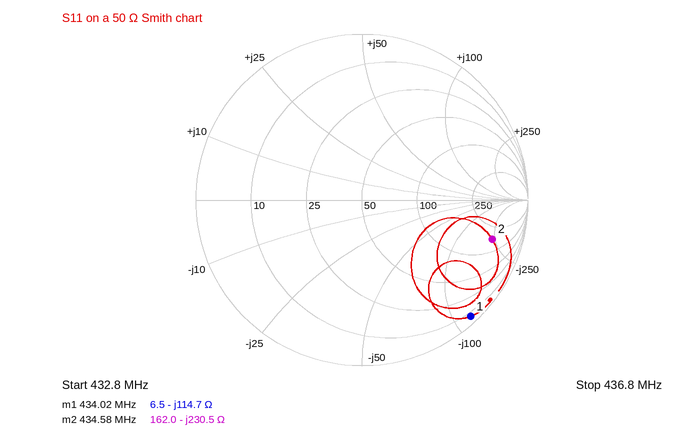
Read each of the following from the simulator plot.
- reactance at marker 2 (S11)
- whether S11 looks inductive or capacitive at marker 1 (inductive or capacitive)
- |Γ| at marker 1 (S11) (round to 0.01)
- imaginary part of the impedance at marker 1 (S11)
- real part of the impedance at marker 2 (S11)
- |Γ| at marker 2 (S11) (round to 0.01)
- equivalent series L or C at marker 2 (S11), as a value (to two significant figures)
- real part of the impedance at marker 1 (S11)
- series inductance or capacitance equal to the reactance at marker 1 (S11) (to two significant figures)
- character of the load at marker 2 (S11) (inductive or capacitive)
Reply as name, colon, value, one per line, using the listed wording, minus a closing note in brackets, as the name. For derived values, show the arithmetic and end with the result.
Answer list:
reactance at marker 2: -230.5 Ω
whether S11 looks inductive or capacitive at marker 1: capacitive
|Γ| at marker 1 (S11): 0.96
imaginary part of the impedance at marker 1: -114.7 Ω
real part of the impedance at marker 2: 162.0 Ω
|Γ| at marker 2 (S11): 0.82
equivalent series L or C at marker 2 (S11), as a value: C = 1/(2π × 434.58 MHz × 230.5 Ω) ≈ 1.6 pF
real part of the impedance at marker 1: 6.5 Ω
series inductance or capacitance equal to the reactance at marker 1 (S11): C = 1/(2π × 434.02 MHz × 114.7 Ω) ≈ 3.2 pF
character of the load at marker 2 (S11): capacitive
